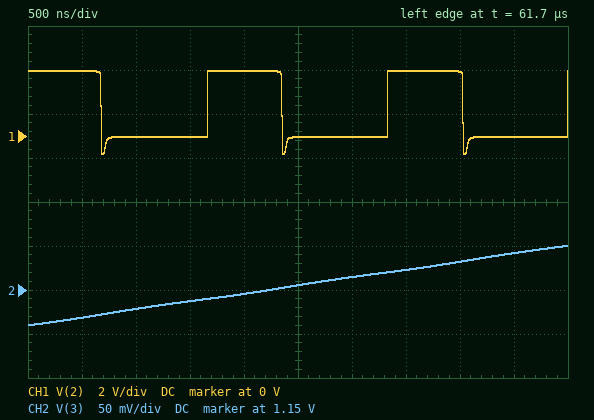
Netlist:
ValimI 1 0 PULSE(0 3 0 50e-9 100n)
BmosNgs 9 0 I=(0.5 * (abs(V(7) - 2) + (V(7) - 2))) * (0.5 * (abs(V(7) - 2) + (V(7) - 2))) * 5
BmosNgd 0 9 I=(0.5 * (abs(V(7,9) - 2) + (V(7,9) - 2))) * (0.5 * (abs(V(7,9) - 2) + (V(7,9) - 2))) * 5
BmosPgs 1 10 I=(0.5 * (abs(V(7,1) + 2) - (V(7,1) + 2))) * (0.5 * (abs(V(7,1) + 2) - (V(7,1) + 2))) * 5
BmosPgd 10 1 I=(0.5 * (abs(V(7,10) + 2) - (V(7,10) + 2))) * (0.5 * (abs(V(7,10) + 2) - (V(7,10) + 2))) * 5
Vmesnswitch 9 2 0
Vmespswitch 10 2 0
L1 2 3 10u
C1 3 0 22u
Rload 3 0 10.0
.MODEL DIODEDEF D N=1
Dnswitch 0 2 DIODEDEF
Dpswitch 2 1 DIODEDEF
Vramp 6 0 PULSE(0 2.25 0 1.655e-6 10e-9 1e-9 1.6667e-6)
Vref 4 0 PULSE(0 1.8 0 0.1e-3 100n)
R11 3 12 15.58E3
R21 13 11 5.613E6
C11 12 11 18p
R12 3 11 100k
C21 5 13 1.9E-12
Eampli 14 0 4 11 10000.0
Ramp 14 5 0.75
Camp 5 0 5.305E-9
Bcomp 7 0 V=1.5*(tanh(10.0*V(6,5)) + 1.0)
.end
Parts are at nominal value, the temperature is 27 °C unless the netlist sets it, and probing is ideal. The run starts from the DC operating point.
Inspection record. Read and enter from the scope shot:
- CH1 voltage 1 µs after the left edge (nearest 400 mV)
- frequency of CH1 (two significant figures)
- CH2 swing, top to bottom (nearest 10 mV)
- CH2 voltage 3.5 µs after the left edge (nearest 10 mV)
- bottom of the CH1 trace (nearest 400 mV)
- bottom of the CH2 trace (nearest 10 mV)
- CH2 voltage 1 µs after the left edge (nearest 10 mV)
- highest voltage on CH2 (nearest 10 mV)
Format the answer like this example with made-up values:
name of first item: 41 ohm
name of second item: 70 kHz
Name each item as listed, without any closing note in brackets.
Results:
CH1 voltage 1 µs after the left edge: 0 V
frequency of CH1: 600 kHz
CH2 swing, top to bottom: 90 mV
CH2 voltage 3.5 µs after the left edge: 1.17 V
bottom of the CH1 trace: -800 mV
bottom of the CH2 trace: 1.11 V
CH2 voltage 1 µs after the left edge: 1.13 V
highest voltage on CH2: 1.20 V
